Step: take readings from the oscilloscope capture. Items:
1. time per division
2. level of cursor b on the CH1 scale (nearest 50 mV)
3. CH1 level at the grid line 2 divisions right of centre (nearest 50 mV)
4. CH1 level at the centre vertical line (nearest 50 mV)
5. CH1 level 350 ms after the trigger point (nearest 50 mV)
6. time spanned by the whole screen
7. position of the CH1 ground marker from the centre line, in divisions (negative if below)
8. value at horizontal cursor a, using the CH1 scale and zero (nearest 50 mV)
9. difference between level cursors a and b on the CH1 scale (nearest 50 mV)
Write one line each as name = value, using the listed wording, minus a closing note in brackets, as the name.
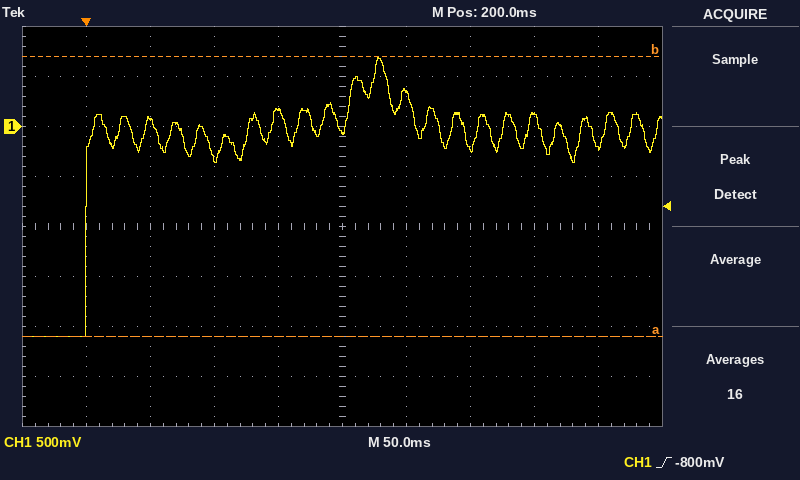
time per division = 50 ms
level of cursor b on the CH1 scale = 700 mV
CH1 level at the grid line 2 divisions right of centre = -200 mV
CH1 level at the centre vertical line = -50 mV
CH1 level 350 ms after the trigger point = 100 mV
time spanned by the whole screen = 500 ms
position of the CH1 ground marker from the centre line, in divisions = +2.0 div
value at horizontal cursor a, using the CH1 scale and zero = -2.10 V
difference between level cursors a and b on the CH1 scale = 2.80 V
